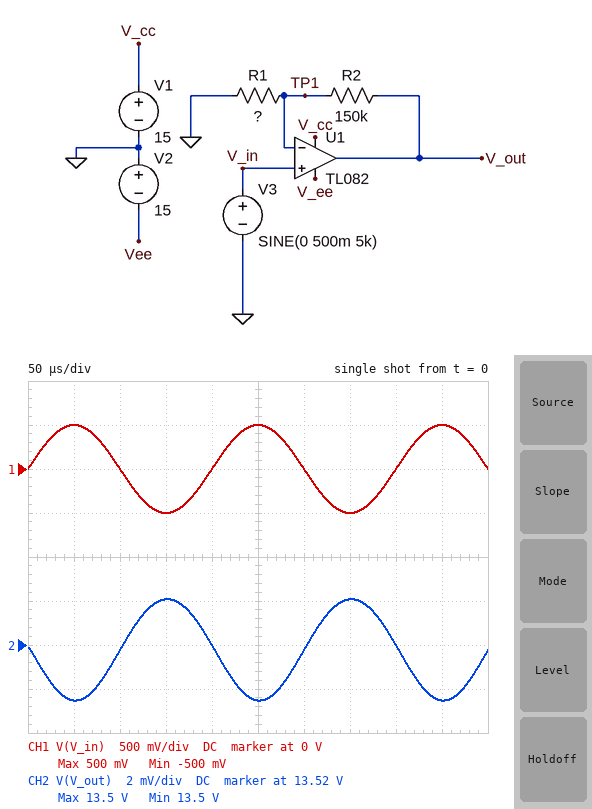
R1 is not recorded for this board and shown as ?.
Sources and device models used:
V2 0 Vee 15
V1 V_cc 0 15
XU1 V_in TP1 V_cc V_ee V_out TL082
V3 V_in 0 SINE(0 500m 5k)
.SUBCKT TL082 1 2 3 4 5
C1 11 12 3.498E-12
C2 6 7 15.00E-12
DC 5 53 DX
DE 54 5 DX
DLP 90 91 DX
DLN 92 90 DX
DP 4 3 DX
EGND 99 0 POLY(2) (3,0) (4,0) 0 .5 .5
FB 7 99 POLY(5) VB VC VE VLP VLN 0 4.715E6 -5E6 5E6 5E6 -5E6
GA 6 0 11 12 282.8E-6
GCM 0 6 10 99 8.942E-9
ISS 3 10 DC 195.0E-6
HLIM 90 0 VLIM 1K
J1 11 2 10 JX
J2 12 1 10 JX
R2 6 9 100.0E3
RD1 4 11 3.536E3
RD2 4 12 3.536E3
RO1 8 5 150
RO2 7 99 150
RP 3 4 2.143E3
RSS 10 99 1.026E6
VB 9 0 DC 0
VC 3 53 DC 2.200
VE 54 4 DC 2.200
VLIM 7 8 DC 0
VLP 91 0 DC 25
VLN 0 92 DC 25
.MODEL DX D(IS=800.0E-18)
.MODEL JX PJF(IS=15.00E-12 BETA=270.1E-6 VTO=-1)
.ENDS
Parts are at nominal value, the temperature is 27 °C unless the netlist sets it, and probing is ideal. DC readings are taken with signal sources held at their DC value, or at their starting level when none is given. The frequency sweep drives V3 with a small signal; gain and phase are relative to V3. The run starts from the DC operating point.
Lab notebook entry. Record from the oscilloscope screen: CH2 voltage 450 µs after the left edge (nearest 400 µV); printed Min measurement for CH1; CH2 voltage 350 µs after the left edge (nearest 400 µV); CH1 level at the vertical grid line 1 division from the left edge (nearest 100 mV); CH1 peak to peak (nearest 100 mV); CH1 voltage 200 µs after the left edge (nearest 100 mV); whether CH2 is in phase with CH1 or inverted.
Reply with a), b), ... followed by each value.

a) 13.5216 V
b) -500 mV
c) 13.5260 V
d) 500 mV
e) 1.0 V
f) 0 V
g) inverted
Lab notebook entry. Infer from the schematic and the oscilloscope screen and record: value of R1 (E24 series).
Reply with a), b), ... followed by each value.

a) 9.1 kΩ
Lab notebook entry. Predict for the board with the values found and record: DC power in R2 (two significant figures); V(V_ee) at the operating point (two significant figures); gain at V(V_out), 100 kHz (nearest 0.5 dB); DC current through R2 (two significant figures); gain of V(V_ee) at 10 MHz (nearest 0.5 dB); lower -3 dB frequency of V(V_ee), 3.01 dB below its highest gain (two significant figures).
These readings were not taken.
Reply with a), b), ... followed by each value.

a) 560 µW
b) 8.2 V
c) -49.5 dB
d) 61 µA
e) -7.5 dB
f) 7.1 MHz
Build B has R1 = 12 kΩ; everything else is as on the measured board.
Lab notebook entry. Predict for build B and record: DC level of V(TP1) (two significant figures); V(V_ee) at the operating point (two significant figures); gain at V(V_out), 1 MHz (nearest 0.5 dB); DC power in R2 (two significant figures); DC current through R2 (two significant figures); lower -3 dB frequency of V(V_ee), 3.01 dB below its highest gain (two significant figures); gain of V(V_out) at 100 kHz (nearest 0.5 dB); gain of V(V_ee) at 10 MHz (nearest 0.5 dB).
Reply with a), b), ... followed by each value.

a) 4.7 V
b) 8.3 V
c) -67.5 dB
d) 520 µW
e) 59 µA
f) 6.2 MHz
g) -50.5 dB
h) -7.5 dB
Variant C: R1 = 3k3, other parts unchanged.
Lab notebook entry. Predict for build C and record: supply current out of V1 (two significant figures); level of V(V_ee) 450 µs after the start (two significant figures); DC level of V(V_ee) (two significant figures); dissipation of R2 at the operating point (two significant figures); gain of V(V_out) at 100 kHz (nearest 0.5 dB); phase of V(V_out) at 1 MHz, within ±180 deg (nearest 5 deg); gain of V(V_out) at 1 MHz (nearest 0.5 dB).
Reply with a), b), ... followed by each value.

a) 2.9 mA
b) 7.9 V
c) 7.8 V
d) 780 µW
e) -44.5 dB
f) 95 deg
g) -61.0 dB
